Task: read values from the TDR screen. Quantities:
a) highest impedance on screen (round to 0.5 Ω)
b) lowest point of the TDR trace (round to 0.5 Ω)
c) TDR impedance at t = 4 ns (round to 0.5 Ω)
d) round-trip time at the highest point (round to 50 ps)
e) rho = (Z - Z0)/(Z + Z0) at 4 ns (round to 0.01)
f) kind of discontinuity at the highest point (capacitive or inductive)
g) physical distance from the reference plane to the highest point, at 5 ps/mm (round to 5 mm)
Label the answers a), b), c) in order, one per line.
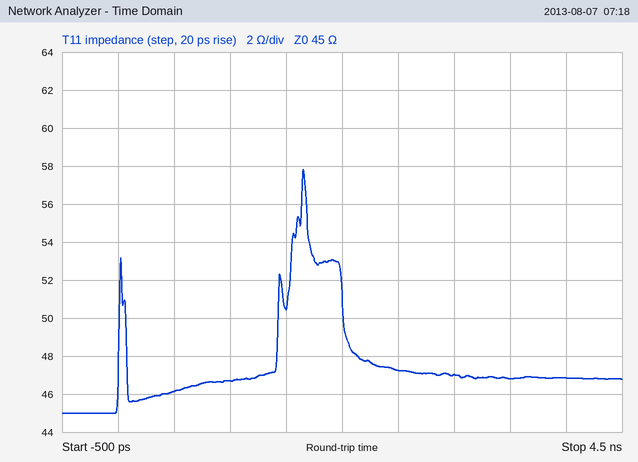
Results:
a) 58.0 Ω
b) 45.0 Ω
c) 47.0 Ω
d) 1.65 ns
e) +0.02
f) inductive
g) 165 mm
